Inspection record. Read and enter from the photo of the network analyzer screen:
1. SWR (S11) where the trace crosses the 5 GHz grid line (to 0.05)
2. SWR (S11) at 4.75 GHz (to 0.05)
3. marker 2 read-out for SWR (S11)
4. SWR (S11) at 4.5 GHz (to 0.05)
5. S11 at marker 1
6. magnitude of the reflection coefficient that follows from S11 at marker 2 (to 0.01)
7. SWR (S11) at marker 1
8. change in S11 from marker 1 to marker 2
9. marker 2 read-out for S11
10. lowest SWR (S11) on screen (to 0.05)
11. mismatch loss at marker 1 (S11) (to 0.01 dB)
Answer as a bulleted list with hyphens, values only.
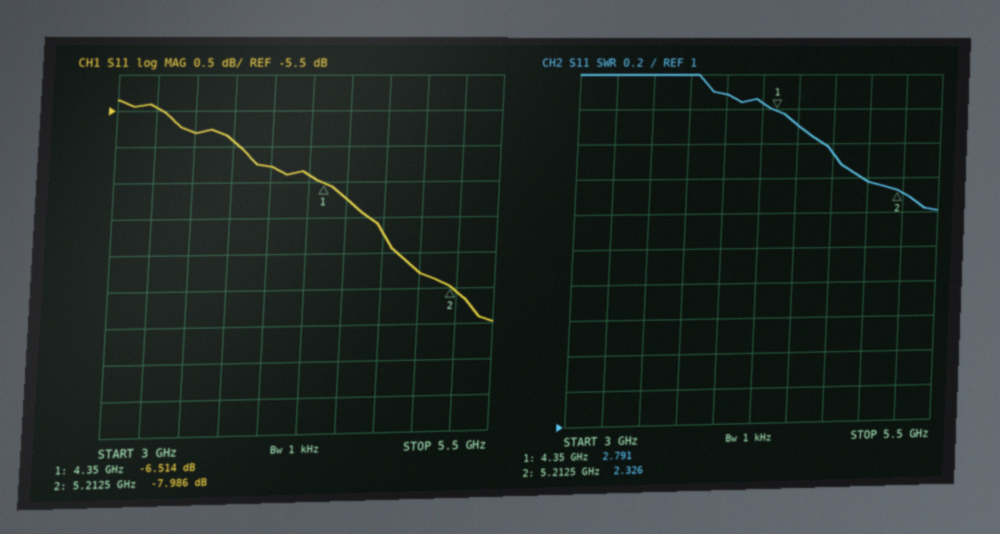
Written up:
- 2.40
- 2.55
- 2.326
- 2.70
- -6.514 dB
- 0.40
- 2.791
- -1.472 dB
- -7.986 dB
- 2.20
- 1.10 dB
